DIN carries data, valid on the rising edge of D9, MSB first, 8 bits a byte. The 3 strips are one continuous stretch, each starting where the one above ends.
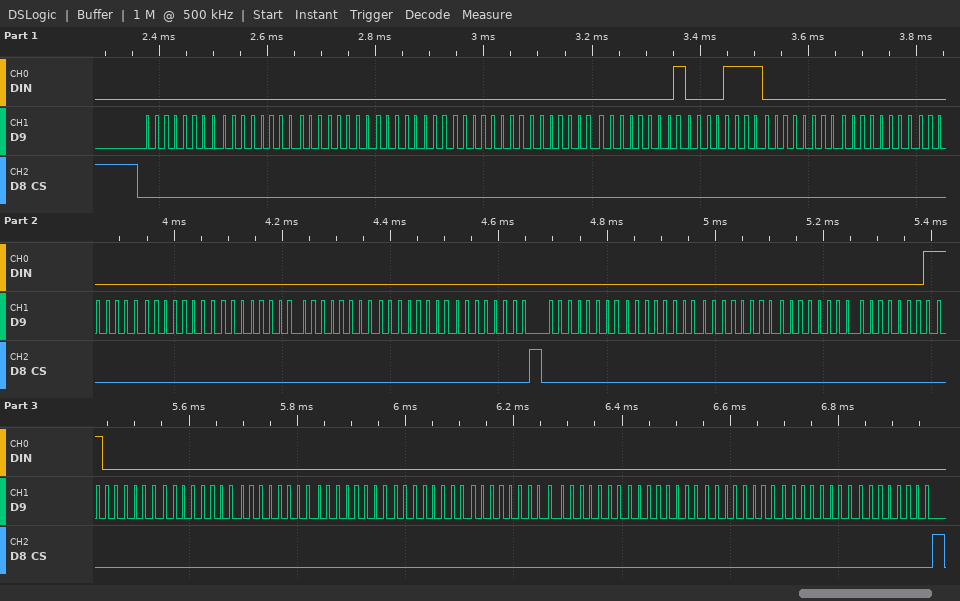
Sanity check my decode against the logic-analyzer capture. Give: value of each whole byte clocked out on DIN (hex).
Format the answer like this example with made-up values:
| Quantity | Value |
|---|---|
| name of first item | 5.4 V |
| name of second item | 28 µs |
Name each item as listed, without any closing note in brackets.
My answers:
| Quantity | Value |
|---|---|
| value of each whole byte clocked out on DIN | 00 00 00 00 00 00 01 0F 00 00 00 00 00 00 00 00 00 00 00 00 01 C0 00 00 00 00 00 00 00 00 00 00 |
